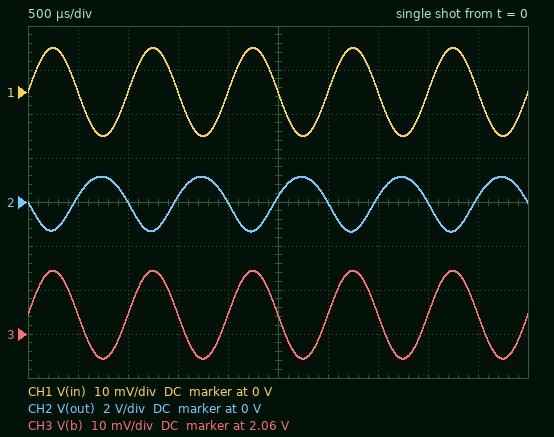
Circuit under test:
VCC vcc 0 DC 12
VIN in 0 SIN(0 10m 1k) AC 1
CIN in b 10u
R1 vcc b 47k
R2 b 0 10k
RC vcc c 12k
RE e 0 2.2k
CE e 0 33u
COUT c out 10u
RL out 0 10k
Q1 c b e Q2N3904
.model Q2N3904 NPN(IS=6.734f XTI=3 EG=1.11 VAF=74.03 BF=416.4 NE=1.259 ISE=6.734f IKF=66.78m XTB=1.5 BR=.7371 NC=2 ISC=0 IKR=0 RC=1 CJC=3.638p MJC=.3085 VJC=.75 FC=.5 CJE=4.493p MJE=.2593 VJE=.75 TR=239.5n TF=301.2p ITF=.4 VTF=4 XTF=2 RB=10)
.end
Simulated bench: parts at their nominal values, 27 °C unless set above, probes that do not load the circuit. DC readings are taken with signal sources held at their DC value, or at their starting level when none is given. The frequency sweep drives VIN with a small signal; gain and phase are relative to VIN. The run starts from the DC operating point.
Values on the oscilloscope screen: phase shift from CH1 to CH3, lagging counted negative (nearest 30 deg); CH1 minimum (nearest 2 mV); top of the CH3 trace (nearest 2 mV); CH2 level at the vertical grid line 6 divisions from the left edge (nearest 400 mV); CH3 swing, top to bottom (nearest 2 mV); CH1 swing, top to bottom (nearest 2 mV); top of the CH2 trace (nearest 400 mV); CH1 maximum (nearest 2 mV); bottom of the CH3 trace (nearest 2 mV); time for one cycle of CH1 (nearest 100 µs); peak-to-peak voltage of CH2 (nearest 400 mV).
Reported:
0 deg
-10 mV
2.074 V
0 V
20 mV
20 mV
1.2 V
10 mV
2.054 V
1.0 ms
2.4 V
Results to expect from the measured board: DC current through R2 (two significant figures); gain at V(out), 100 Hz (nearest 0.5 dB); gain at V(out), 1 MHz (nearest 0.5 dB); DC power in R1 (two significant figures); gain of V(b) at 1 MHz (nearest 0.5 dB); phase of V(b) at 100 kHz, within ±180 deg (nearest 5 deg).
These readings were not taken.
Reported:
210 µA
38.5 dB
42.0 dB
2.1 mW
0 dB
0 deg
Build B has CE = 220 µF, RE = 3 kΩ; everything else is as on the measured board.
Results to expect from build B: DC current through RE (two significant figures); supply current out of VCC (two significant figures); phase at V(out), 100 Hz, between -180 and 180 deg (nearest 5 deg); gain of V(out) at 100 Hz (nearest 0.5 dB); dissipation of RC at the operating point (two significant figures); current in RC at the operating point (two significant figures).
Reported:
480 µA
680 µA
-170 deg
39.5 dB
2.7 mW
470 µA
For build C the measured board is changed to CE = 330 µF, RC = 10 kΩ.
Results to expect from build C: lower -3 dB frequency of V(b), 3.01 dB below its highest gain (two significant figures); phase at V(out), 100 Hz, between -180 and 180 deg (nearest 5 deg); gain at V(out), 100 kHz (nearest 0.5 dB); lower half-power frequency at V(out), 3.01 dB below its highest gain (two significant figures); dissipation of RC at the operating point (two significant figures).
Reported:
2.9 Hz
-170 deg
41.5 dB
15 Hz
4.1 mW
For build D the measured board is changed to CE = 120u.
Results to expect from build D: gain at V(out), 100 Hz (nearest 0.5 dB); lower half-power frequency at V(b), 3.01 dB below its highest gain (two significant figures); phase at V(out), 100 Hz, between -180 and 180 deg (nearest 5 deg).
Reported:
41.5 dB
2.2 Hz
-160 deg
